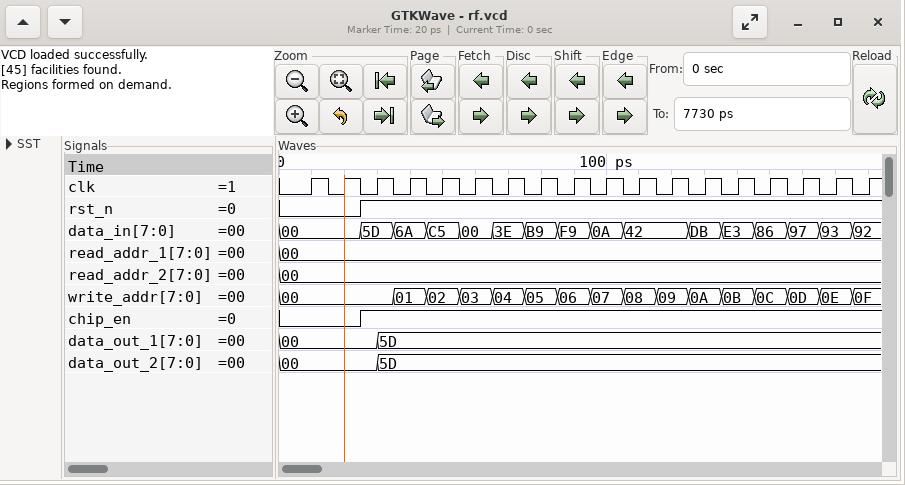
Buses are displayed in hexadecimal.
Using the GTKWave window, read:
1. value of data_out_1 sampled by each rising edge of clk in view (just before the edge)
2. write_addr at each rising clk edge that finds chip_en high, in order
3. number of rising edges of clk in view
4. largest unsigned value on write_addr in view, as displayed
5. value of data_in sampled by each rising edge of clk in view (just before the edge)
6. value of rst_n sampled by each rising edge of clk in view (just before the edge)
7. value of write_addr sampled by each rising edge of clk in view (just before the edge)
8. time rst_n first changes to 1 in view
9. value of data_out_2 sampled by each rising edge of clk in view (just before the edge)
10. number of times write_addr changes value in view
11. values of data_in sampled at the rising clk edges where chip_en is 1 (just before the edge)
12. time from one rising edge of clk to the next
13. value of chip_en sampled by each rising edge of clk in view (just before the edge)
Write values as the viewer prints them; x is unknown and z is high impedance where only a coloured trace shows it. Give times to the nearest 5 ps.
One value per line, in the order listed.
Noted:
00, 00, 00, 5D, 5D, 5D, 5D, 5D, 5D, 5D, 5D, 5D, 5D, 5D, 5D, 5D, 5D, 5D
00, 01, 02, 03, 04, 05, 06, 07, 08, 09, 0A, 0B, 0C, 0D, 0E, 0F
18
0F
00, 00, 5D, 6A, C5, 00, 3E, B9, F9, 0A, 42, 42, DB, E3, 86, 97, 93, 92
0 0 1 1 1 1 1 1 1 1 1 1 1 1 1 1 1 1
00, 00, 00, 01, 02, 03, 04, 05, 06, 07, 08, 09, 0A, 0B, 0C, 0D, 0E, 0F
25 ps
00, 00, 00, 5D, 5D, 5D, 5D, 5D, 5D, 5D, 5D, 5D, 5D, 5D, 5D, 5D, 5D, 5D
15
5D, 6A, C5, 00, 3E, B9, F9, 0A, 42, 42, DB, E3, 86, 97, 93, 92
10 ps
0 0 1 1 1 1 1 1 1 1 1 1 1 1 1 1 1 1
